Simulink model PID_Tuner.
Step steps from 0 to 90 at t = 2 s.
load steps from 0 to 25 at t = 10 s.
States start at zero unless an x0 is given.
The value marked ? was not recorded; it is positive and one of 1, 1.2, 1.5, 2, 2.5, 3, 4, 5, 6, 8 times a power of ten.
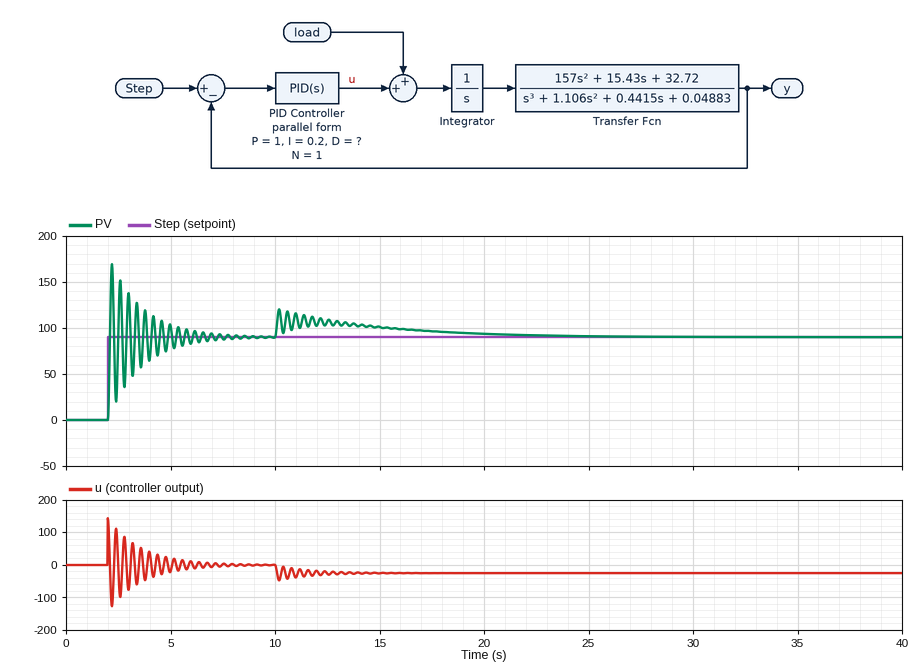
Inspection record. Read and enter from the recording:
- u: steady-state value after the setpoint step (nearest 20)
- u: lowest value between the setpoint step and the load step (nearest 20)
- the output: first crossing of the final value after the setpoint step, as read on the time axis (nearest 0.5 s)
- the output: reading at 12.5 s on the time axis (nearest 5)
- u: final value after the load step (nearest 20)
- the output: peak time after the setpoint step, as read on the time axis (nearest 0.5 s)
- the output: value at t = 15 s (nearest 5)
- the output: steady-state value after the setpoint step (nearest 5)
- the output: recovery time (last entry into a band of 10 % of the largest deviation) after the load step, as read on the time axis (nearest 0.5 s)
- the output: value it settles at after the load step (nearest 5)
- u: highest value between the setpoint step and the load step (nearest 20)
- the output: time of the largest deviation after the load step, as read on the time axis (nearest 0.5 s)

0
-120
2.0 s
105
-20
2.0 s
100
90
21.0 s
90
140
10.0 s
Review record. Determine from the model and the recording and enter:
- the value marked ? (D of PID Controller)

0.6
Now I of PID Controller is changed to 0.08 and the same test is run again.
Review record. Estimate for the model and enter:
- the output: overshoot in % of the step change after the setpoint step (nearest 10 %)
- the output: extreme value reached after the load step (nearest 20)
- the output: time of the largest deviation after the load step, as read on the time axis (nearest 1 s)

90 %
120
10 s
